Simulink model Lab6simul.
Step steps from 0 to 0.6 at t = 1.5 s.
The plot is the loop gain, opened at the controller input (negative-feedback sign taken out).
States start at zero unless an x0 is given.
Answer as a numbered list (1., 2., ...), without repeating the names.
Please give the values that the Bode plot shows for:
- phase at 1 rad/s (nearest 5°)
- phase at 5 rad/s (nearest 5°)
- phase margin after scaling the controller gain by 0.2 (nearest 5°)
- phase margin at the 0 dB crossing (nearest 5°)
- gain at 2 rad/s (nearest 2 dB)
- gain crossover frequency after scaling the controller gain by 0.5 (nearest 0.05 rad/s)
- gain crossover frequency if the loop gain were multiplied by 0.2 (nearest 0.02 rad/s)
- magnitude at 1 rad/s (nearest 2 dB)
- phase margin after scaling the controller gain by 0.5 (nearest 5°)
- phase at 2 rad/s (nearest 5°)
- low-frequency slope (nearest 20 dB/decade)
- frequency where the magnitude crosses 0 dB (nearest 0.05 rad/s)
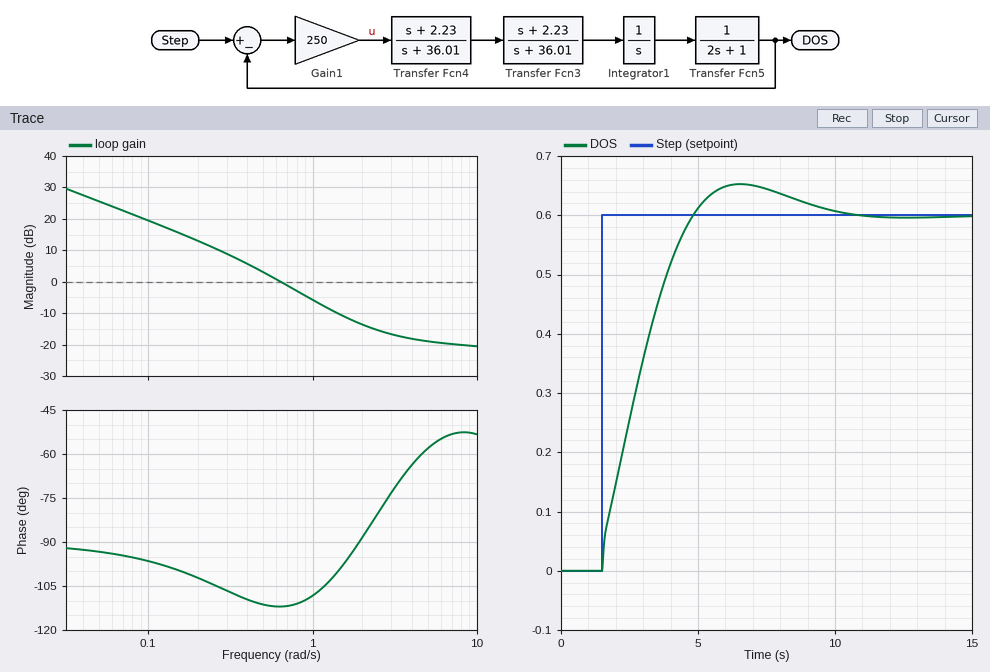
1. -110°
2. -60°
3. 80°
4. 70°
5. -14 dB
6. 0.40 rad/s
7. 0.18 rad/s
8. -6 dB
9. 70°
10. -90°
11. -20 dB/decade
12. 0.65 rad/s
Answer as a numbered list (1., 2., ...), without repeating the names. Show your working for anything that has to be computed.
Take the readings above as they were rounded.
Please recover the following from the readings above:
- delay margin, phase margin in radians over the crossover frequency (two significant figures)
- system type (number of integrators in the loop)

1. 70 × π / 180 / 0.65 = 1.9 s
2. 1
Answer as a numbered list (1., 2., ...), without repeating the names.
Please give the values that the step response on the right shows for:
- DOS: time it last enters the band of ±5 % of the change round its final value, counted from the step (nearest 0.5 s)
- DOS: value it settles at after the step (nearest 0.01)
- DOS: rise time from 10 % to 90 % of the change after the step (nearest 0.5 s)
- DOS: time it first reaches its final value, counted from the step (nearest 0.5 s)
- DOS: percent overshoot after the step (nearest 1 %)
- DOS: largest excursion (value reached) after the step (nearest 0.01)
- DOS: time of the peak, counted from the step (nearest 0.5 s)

1. 7.0 s
2. 0.60
3. 2.5 s
4. 3.5 s
5. 9 %
6. 0.65
7. 5.0 s
